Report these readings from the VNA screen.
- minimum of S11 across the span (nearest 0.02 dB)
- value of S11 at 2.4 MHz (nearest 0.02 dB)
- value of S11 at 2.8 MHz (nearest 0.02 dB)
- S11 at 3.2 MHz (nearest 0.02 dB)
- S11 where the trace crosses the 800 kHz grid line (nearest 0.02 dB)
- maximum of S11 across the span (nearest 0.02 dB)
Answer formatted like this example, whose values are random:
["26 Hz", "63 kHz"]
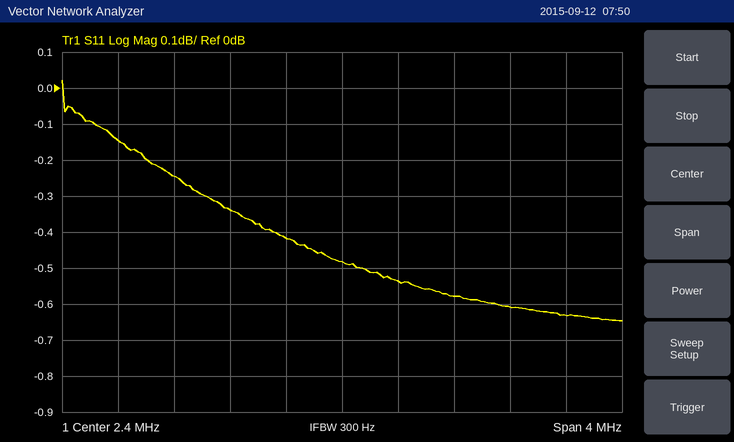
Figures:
["-0.64 dB", "-0.48 dB", "-0.54 dB", "-0.58 dB", "-0.14 dB", "0.02 dB"]
